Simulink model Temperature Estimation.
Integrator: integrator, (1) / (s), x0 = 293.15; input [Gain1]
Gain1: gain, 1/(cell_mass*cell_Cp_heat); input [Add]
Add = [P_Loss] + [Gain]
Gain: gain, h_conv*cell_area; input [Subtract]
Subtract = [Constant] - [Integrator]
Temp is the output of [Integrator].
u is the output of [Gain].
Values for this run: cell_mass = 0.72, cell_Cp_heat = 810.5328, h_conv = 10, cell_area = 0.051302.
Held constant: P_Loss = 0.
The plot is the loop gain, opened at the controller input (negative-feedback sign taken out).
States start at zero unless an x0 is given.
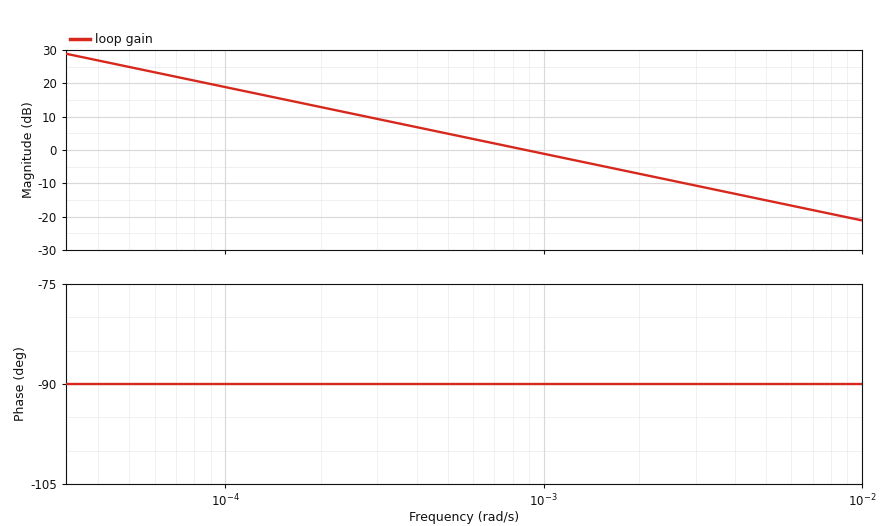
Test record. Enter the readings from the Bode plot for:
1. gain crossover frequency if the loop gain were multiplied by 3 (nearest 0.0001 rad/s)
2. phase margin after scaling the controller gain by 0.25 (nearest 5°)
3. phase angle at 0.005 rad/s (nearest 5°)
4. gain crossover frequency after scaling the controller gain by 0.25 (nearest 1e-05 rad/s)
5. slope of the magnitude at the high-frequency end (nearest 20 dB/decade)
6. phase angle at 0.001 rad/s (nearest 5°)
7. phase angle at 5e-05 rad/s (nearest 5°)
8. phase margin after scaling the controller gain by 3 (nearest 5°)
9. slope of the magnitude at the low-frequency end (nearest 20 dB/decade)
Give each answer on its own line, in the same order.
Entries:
0.0026 rad/s
90°
-90°
0.00022 rad/s
-20 dB/decade
-90°
-90°
90°
-20 dB/decade
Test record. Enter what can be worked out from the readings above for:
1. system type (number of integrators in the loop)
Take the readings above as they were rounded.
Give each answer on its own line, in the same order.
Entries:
1
